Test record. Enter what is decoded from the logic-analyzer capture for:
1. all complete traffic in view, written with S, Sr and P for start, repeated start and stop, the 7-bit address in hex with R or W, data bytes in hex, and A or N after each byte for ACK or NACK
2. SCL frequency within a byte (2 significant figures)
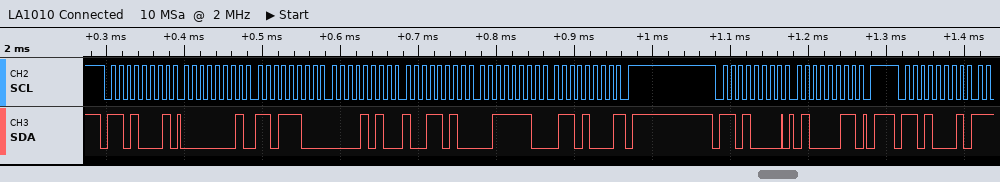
S 68R A 01 A DC A 0A A 9A A 3E A 68 N P S 68W A 43 A P S 68R A
100 kHz
